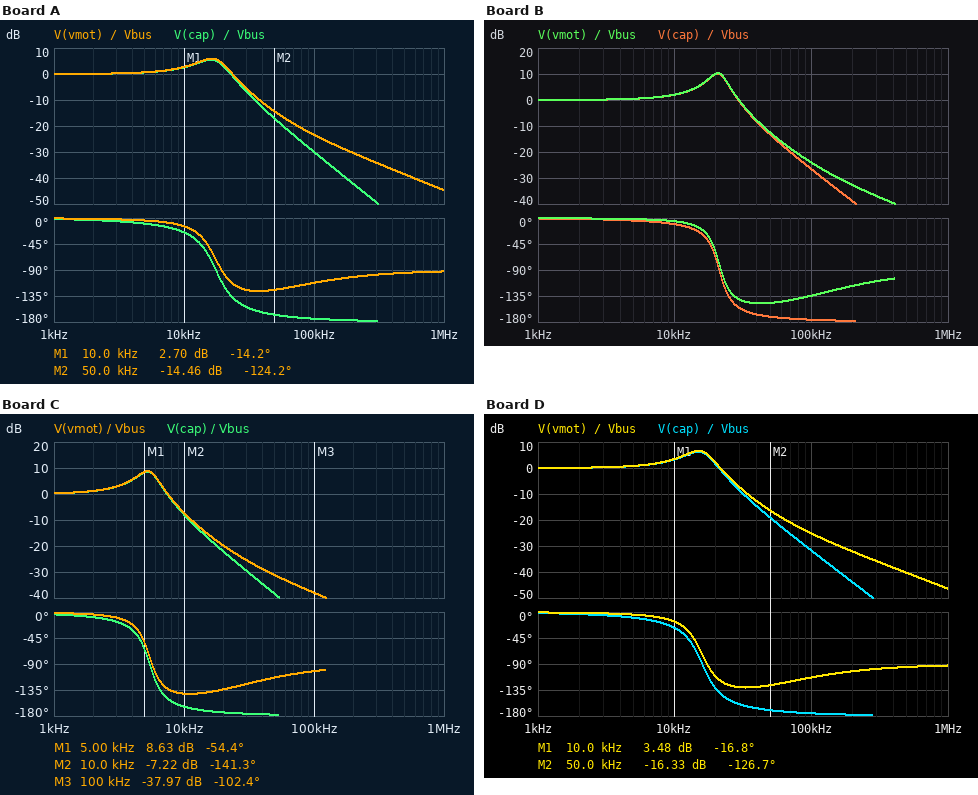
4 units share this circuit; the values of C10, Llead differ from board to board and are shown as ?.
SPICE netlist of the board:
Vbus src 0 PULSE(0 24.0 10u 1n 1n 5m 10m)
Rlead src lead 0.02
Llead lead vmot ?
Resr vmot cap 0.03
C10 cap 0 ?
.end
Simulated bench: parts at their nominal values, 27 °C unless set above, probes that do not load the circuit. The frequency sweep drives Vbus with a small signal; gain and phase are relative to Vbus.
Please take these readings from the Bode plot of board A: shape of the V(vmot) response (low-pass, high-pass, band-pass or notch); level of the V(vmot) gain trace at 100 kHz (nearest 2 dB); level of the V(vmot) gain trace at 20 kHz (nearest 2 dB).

low-pass
-24 dB
4 dB
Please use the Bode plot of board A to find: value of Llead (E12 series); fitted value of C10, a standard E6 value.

820 nH
100 µF
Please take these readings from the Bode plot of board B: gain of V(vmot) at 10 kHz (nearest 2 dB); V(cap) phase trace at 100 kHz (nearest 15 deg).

2 dB
-180 deg
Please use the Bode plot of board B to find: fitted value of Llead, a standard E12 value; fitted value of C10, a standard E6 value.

1.2 µH
47 µF
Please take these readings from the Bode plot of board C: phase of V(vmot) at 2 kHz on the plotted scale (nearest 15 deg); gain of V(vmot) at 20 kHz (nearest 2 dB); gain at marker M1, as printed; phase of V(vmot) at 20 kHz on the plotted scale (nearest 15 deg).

0 deg
-20 dB
8.63 dB
-135 deg
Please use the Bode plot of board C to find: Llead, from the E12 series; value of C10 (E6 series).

3.9 µH
220 µF
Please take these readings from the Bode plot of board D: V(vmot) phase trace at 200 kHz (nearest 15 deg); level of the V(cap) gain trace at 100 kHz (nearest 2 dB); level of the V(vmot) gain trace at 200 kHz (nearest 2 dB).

-105 deg
-32 dB
-32 dB
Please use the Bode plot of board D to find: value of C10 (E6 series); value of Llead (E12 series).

100 µF
1 µH
